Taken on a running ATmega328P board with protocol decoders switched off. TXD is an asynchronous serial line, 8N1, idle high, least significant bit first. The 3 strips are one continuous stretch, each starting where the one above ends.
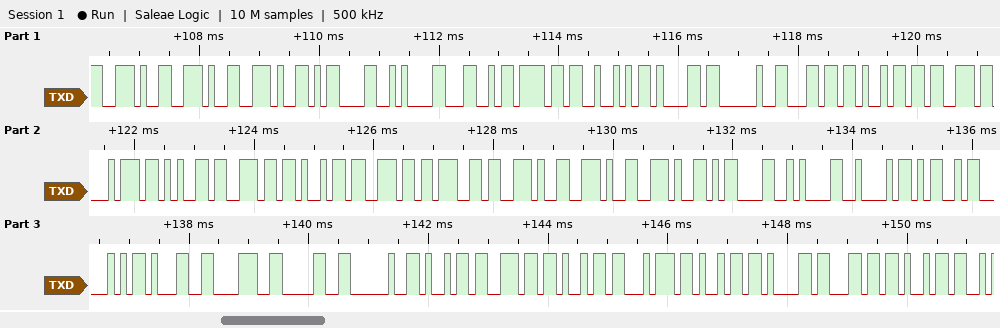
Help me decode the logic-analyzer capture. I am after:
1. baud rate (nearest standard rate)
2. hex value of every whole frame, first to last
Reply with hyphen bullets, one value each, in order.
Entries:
- 9600 baud
- 2E 2E 2E 0D 0A 4C 6F 52 61 20 6C 69 73 74 65 6E 69 6E 67 2E 2E 2E 0D 0A 42 4D 50 31 38 30 20 69 6E 69 74 69 61 6C 69
